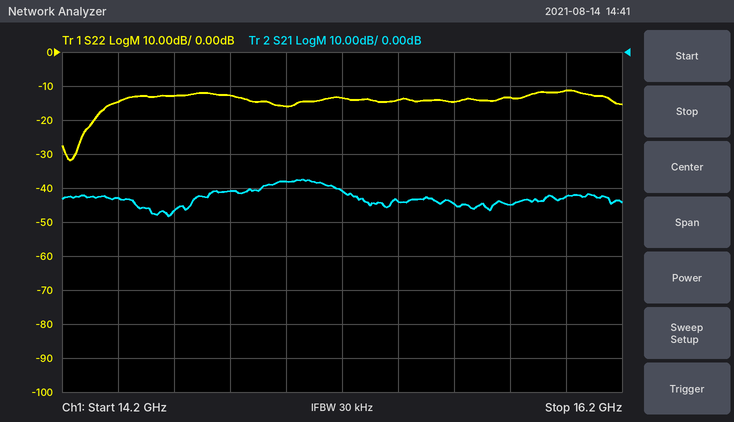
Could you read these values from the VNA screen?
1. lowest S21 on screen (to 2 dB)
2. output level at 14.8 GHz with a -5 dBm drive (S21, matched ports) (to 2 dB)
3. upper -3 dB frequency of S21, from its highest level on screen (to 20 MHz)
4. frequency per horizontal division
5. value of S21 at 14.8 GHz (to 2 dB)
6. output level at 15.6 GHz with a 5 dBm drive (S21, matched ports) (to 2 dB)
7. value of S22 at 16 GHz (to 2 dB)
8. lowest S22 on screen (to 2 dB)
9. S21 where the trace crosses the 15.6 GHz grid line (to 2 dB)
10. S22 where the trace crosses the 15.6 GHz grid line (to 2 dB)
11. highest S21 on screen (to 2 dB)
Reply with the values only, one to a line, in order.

-48 dB
-46 dBm
15.20 GHz
200 MHz
-40 dB
-40 dBm
-12 dB
-32 dB
-44 dB
-14 dB
-38 dB
